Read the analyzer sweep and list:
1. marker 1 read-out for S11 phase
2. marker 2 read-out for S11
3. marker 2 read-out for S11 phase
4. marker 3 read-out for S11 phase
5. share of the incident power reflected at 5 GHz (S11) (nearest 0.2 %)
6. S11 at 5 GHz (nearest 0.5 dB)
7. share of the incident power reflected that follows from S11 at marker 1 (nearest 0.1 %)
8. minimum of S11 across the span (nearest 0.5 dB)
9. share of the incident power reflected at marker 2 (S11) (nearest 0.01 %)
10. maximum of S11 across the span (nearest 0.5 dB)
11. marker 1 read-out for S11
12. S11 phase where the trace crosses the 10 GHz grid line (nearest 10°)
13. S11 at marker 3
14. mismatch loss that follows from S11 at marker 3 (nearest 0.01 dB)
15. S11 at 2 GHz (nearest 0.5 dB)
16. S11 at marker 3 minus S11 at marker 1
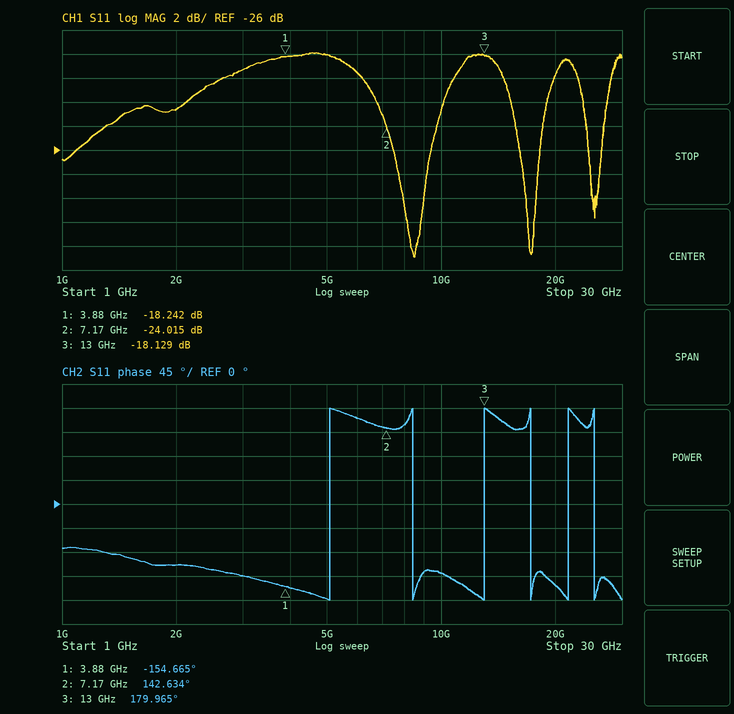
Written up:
-154.665°
-24.015 dB
142.634°
179.965°
1.6 %
-18.0 dB
1.5 %
-35.0 dB
0.40 %
-18.0 dB
-18.242 dB
-130°
-18.129 dB
0.07 dB
-22.5 dB
0.113 dB
